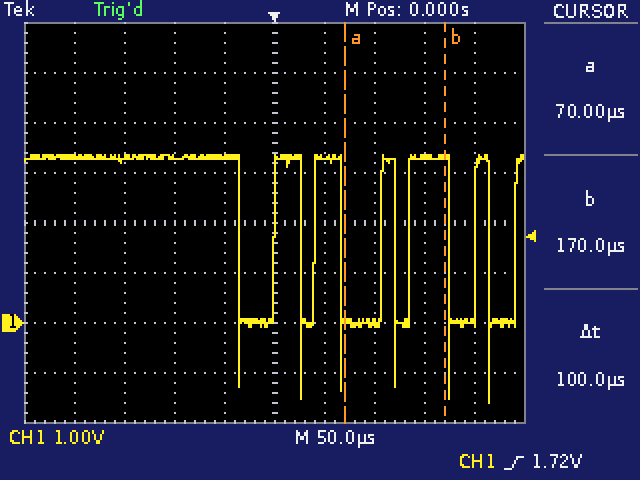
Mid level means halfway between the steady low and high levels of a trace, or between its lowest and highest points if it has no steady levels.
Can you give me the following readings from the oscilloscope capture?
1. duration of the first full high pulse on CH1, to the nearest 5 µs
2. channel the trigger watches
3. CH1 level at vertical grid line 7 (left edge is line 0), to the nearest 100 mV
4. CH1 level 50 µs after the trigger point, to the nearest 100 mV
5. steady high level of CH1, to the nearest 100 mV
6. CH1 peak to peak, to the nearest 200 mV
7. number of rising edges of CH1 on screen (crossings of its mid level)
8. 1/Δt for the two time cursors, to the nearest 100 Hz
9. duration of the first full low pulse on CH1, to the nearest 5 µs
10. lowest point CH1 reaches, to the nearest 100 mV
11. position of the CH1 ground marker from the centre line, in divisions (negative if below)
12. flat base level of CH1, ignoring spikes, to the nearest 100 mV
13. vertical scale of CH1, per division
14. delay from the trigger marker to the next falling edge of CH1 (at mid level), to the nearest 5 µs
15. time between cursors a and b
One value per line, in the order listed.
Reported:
25 µs
CH1
0.0 V
3.3 V
3.3 V
5.0 V
6
10.0 kHz
35 µs
-1.6 V
-2.0 div
0.0 V
1 V
25 µs
100 µs
